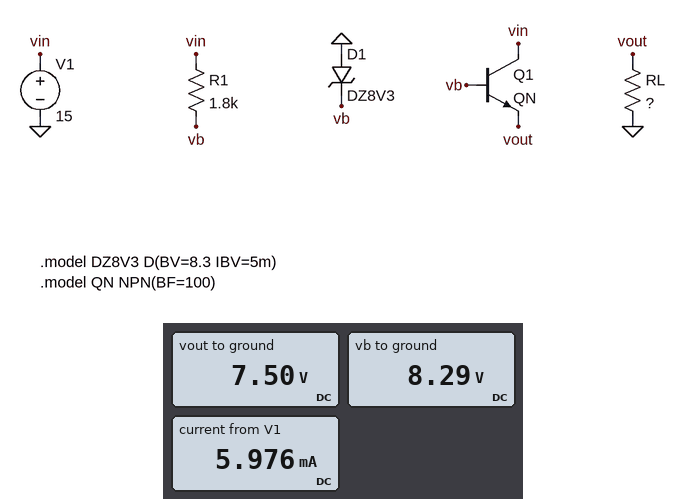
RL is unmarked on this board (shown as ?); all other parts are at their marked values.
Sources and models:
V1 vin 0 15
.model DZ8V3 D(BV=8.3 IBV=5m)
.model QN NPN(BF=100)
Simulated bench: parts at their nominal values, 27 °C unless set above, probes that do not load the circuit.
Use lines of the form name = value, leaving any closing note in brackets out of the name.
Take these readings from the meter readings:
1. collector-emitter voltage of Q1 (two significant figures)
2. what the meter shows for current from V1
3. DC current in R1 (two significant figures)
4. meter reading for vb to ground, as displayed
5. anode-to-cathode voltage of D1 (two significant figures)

collector-emitter voltage of Q1 = 7.5 V
what the meter shows for current from V1 = 5.976 mA
DC current in R1 = 3.7 mA
meter reading for vb to ground, as displayed = 8.29 V
anode-to-cathode voltage of D1 = -8.3 V
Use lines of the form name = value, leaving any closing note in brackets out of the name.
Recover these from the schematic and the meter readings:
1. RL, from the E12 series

RL, from the E12 series = 3.3 kΩ
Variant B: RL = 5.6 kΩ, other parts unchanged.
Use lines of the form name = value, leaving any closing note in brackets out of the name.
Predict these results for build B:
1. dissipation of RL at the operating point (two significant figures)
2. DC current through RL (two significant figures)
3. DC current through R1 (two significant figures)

dissipation of RL at the operating point = 10 mW
DC current through RL = 1.3 mA
DC current through R1 = 3.7 mA
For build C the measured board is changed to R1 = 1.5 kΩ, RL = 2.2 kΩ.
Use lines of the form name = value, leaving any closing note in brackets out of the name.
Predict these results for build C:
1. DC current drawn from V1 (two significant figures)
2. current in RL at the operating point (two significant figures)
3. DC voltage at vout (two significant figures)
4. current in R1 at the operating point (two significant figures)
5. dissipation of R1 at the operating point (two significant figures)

DC current drawn from V1 = 7.8 mA
current in RL at the operating point = 3.4 mA
DC voltage at vout = 7.5 V
current in R1 at the operating point = 4.5 mA
dissipation of R1 at the operating point = 30 mW
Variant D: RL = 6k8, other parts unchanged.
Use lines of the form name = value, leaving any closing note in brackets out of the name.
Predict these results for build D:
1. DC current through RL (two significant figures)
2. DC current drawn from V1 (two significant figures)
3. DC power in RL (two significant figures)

DC current through RL = 1.1 mA
DC current drawn from V1 = 4.8 mA
DC power in RL = 8.3 mW
